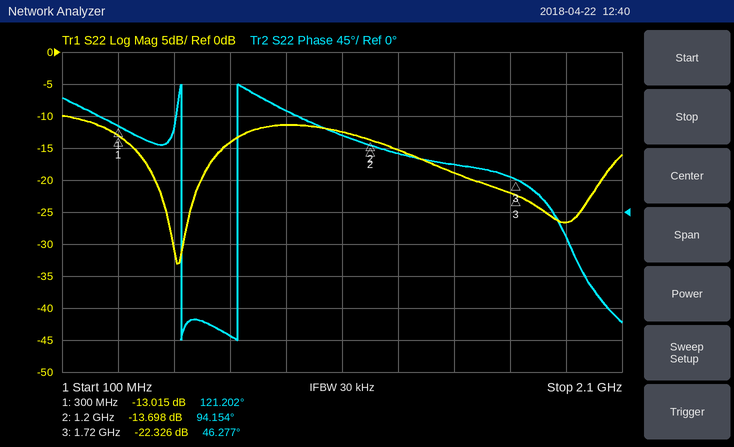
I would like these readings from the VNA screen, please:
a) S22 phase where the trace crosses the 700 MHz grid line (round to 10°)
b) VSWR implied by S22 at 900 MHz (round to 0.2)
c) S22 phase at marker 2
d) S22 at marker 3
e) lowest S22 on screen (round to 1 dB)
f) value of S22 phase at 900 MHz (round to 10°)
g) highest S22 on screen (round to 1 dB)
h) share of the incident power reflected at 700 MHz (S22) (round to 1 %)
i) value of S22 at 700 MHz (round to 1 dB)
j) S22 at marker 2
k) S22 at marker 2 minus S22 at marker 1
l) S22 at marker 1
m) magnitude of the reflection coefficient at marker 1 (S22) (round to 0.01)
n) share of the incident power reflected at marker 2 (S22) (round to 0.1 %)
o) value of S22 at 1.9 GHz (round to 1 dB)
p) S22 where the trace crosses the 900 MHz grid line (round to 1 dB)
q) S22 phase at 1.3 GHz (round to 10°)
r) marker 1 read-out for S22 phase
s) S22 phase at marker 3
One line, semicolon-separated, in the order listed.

-170°; 1.8; 94.154°; -22.326 dB; -33 dB; 140°; -10 dB; 4 %; -14 dB; -13.698 dB; -0.683 dB; -13.015 dB; 0.22; 4.3 %; -27 dB; -11 dB; 80°; 121.202°; 46.277°
